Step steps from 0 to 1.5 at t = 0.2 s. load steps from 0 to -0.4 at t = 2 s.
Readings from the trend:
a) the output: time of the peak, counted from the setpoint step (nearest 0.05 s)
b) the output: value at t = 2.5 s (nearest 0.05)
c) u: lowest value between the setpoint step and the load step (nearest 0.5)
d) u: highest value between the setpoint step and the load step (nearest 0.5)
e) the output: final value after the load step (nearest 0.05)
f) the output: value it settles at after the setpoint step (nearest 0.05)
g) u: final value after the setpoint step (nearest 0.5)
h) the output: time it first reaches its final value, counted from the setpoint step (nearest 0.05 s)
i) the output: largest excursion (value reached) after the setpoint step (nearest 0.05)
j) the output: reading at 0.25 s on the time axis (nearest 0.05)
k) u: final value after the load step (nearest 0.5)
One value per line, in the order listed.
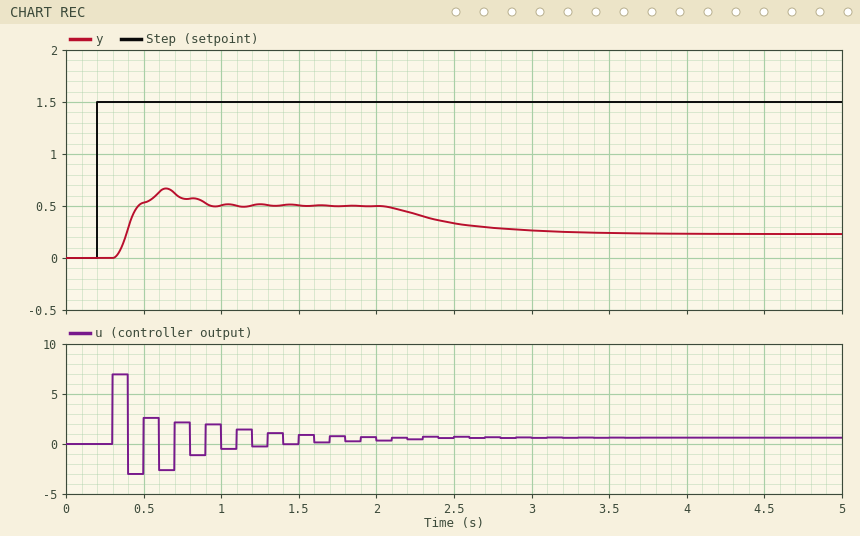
0.45 s
0.35
-3.0
7.0
0.25
0.50
0.5
0.25 s
0.65
0.00
0.5
